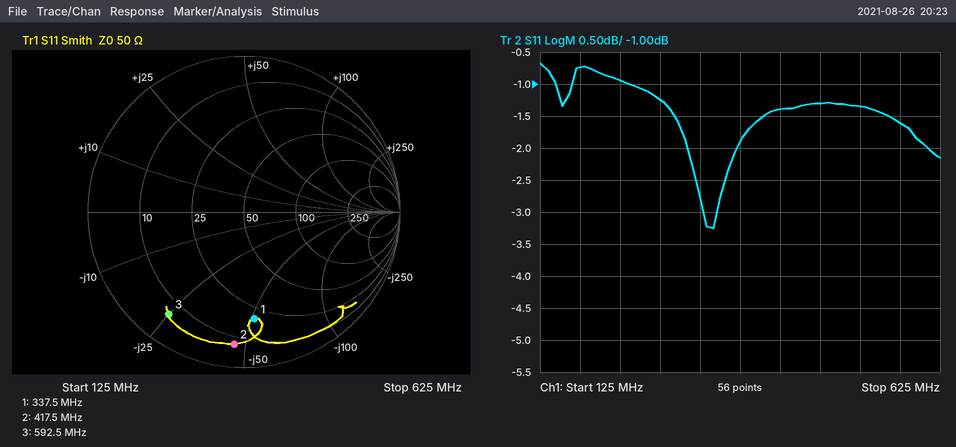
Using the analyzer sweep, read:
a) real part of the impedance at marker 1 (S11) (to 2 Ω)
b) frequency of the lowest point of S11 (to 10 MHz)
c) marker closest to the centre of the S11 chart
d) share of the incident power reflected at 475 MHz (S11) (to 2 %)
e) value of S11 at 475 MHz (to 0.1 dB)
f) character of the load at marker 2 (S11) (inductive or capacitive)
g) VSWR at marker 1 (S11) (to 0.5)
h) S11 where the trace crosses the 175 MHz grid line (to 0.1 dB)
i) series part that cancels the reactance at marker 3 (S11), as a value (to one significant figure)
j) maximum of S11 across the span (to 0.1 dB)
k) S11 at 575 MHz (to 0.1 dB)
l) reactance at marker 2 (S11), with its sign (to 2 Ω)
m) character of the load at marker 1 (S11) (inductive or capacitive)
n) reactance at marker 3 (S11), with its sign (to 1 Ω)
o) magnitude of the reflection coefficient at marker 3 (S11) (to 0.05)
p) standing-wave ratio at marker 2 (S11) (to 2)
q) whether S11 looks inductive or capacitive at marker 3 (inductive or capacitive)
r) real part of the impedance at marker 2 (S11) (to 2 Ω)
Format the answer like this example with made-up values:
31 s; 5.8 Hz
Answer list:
20 Ω; 340 MHz; marker 1; 74 %; -1.3 dB; capacitive; 5.5; -0.7 dB; 7 nH; -0.7 dB; -1.6 dB; -46 Ω; capacitive; -25 Ω; 0.80; 12; capacitive; 8 Ω
